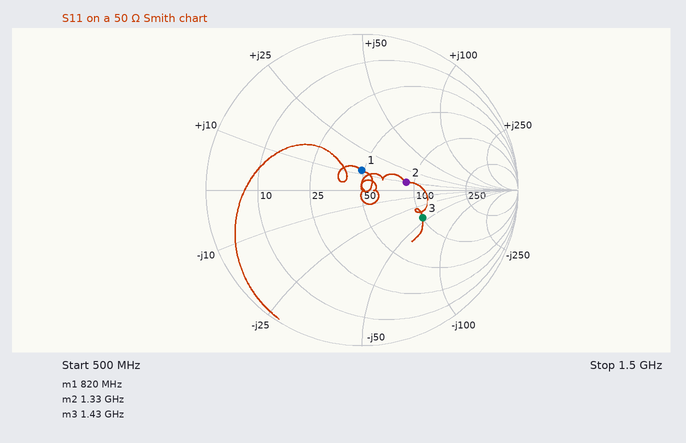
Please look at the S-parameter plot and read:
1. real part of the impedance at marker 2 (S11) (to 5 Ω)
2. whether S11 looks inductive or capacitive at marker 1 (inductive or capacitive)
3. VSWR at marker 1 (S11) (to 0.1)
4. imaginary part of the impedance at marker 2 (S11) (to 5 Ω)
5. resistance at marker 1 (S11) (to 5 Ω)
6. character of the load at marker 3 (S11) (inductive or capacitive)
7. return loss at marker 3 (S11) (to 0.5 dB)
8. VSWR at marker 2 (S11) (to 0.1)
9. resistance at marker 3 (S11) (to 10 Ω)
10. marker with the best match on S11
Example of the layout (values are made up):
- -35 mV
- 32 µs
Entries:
- 90 Ω
- inductive
- 1.3
- +10 Ω
- 50 Ω
- capacitive
- 7.5 dB
- 1.8
- 100 Ω
- marker 1
